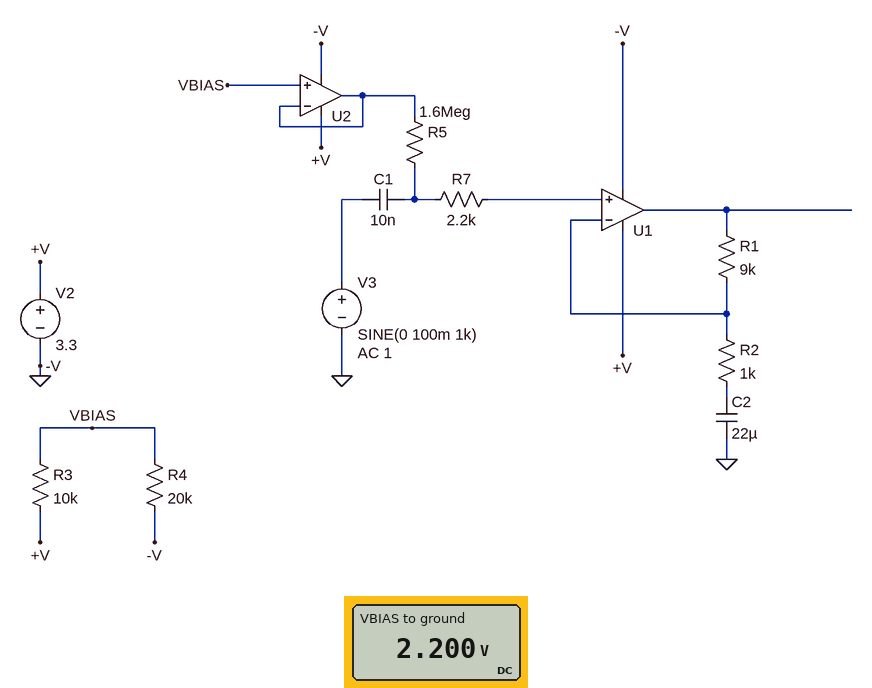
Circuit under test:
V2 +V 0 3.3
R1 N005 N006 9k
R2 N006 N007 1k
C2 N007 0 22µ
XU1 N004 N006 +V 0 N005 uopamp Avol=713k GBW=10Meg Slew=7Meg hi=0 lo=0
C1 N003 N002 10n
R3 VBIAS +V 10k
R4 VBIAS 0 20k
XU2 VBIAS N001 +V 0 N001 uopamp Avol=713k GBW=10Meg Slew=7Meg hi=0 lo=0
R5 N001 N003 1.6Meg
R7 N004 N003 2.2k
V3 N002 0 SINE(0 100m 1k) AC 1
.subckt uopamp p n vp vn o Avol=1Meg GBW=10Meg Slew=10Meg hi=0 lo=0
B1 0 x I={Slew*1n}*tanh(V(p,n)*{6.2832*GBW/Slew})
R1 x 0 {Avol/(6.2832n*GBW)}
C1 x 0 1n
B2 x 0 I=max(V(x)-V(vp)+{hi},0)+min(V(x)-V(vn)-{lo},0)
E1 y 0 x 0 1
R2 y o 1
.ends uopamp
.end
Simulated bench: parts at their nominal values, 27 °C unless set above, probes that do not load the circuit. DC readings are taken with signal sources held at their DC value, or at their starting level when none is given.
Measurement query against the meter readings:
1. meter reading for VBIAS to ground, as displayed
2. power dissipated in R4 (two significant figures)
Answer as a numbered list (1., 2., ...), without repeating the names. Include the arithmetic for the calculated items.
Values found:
1. 2.200 V
2. (2.2 V)^2 / 20 kΩ = 240 µW
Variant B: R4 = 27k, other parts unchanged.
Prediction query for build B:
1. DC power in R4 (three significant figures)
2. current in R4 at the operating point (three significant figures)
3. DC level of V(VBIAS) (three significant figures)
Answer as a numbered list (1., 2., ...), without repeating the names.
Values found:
1. 215 µW
2. 89.2 µA
3. 2.41 V
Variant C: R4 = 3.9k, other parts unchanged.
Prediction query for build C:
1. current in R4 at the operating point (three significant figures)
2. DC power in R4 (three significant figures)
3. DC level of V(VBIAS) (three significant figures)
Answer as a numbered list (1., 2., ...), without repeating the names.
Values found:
1. 237 µA
2. 220 µW
3. 926 mV
